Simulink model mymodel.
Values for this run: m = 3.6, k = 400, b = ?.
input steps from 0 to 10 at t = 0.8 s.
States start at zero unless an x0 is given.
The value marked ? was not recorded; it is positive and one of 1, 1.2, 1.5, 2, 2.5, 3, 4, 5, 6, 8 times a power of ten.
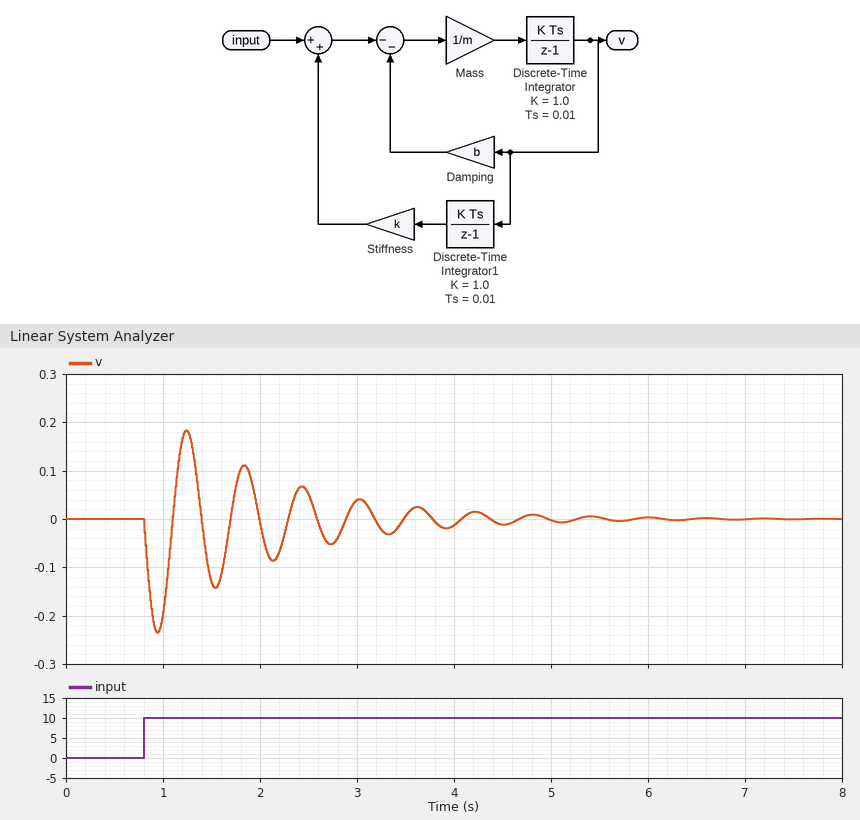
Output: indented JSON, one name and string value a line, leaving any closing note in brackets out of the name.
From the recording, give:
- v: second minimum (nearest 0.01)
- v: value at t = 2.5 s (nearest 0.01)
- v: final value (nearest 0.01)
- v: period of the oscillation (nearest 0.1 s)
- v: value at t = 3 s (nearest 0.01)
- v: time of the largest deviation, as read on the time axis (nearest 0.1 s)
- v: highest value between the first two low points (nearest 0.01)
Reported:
{
  "v: second minimum": "-0.14",
  "v: value at t = 2.5 s": "0.05",
  "v: final value": "0.00",
  "v: period of the oscillation": "0.6 s",
  "v: value at t = 3 s": "0.04",
  "v: time of the largest deviation, as read on the time axis": "0.9 s",
  "v: highest value between the first two low points": "0.18"
}
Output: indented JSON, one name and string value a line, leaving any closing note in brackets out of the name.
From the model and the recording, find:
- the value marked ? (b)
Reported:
{
  "the value marked ?": "10"
}
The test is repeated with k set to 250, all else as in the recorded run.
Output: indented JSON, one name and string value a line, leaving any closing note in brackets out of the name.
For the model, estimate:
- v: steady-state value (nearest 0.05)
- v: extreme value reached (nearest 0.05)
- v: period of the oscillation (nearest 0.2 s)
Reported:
{
  "v: steady-state value": "0.00",
  "v: extreme value reached": "-0.30",
  "v: period of the oscillation": "0.8 s"
}
